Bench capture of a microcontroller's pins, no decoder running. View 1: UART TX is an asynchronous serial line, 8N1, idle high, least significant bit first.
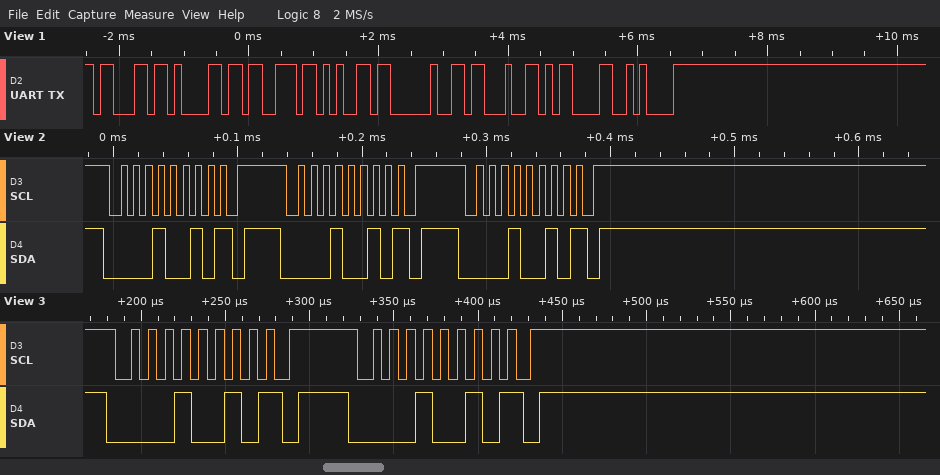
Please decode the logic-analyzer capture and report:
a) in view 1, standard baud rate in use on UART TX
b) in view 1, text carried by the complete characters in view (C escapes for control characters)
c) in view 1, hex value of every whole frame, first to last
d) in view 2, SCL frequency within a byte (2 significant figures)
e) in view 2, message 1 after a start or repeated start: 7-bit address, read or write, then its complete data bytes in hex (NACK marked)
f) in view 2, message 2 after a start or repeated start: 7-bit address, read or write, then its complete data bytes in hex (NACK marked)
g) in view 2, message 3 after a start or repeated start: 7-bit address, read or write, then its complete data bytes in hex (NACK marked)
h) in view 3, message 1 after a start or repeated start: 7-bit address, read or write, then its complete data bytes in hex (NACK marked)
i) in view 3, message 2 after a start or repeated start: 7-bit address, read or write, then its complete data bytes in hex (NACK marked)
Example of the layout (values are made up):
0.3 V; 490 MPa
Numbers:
9600 baud; "case #\r\n"; 63 61 73 65 20 23 0D 0A; 100 kHz; 0x09 write NACK; 0x09 write NACK; 0x09 write NACK; 0x09 write NACK; 0x09 write NACK
